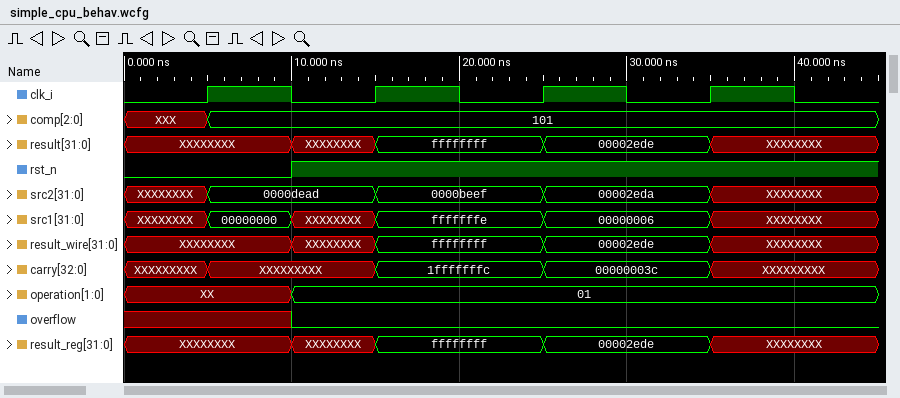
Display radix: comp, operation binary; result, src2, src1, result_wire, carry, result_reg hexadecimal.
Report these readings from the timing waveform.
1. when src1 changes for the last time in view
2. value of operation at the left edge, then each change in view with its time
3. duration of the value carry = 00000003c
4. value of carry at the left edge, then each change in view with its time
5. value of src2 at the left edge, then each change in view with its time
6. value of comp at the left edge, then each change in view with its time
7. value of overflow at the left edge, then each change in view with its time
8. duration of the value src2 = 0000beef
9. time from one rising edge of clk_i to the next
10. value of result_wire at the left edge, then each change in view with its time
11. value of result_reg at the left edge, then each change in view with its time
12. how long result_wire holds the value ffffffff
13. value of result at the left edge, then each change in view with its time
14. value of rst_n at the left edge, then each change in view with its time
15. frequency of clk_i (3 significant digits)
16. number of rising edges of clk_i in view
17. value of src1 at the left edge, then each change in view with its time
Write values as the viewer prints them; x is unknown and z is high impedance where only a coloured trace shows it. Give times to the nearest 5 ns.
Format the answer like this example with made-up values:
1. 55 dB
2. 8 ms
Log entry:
1. 35 ns
2. XX, 01 at 10 ns
3. 10 ns
4. XXXXXXXXX, XXXXXXXXX at 5 ns, 1fffffffc at 15 ns, 00000003c at 25 ns, XXXXXXXXX at 35 ns
5. XXXXXXXX, 0000dead at 5 ns, 0000beef at 15 ns, 00002eda at 25 ns, XXXXXXXX at 35 ns
6. XXX, 101 at 5 ns
7. x, 0 at 10 ns
8. 10 ns
9. 10 ns
10. XXXXXXXX, XXXXXXXX at 10 ns, ffffffff at 15 ns, 00002ede at 25 ns, XXXXXXXX at 35 ns
11. XXXXXXXX, XXXXXXXX at 10 ns, ffffffff at 15 ns, 00002ede at 25 ns, XXXXXXXX at 35 ns
12. 10 ns
13. XXXXXXXX, XXXXXXXX at 10 ns, ffffffff at 15 ns, 00002ede at 25 ns, XXXXXXXX at 35 ns
14. 0, 1 at 10 ns
15. 100 MHz
16. 4
17. XXXXXXXX, 00000000 at 5 ns, XXXXXXXX at 10 ns, fffffffe at 15 ns, 00000006 at 25 ns, XXXXXXXX at 35 ns
